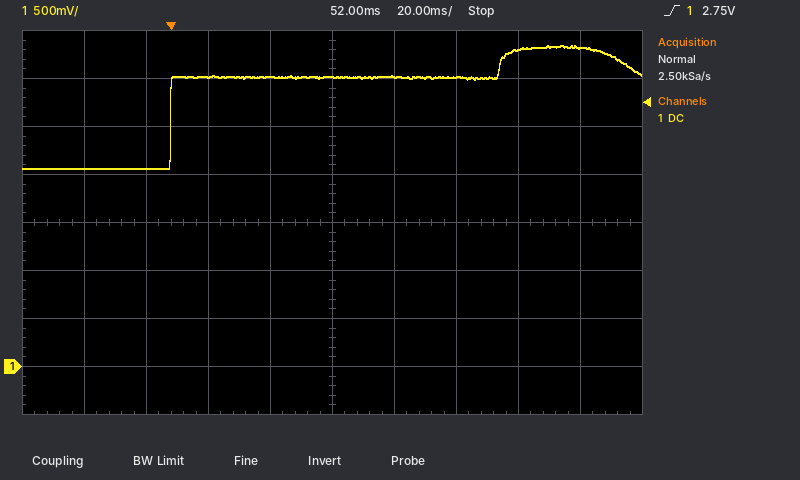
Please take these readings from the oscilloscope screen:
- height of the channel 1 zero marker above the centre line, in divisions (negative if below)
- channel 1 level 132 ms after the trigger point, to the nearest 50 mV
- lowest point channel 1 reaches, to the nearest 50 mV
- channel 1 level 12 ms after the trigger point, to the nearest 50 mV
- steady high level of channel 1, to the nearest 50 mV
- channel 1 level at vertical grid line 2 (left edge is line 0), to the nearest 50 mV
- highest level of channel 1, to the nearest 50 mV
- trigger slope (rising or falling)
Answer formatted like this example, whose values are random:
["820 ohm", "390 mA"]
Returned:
["-3.0 div", "3.30 V", "2.05 V", "3.00 V", "3.00 V", "2.05 V", "3.35 V", "rising"]
